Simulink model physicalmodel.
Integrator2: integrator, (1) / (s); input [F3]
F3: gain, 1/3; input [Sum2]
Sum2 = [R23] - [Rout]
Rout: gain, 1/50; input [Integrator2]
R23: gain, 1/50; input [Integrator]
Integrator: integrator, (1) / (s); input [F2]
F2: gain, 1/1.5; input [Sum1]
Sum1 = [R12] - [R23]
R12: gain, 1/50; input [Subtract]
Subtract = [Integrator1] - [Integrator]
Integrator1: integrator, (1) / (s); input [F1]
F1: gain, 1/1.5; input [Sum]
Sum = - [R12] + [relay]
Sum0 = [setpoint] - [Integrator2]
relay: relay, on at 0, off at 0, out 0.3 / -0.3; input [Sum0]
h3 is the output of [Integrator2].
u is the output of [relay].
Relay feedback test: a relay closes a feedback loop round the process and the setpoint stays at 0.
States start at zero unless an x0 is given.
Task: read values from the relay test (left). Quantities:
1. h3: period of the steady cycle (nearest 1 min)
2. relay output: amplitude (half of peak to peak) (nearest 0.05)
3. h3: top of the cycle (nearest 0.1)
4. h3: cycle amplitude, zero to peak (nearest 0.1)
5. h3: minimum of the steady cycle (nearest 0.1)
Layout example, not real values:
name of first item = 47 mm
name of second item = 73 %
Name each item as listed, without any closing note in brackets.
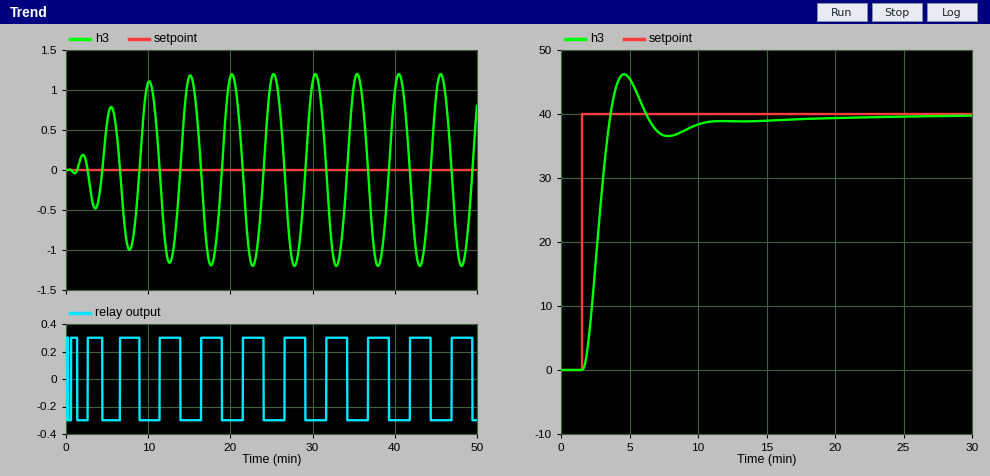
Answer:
h3: period of the steady cycle = 5 min
relay output: amplitude (half of peak to peak) = 0.30
h3: top of the cycle = 1.2
h3: cycle amplitude, zero to peak = 1.2
h3: minimum of the steady cycle = -1.2
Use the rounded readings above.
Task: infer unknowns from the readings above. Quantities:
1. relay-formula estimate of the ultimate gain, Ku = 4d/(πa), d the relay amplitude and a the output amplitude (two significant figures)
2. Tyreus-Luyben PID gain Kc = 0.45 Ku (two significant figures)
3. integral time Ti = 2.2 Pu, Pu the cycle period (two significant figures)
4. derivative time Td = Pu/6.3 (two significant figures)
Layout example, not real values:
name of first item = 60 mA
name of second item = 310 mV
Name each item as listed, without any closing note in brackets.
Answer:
relay-formula estimate of the ultimate gain, Ku = 4d/(πa), d the relay amplitude and a the output amplitude = 0.32
Tyreus-Luyben PID gain Kc = 0.45 Ku = 0.14
integral time Ti = 2.2 Pu, Pu the cycle period = 11 min
derivative time Td = Pu/6.3 = 0.79 min
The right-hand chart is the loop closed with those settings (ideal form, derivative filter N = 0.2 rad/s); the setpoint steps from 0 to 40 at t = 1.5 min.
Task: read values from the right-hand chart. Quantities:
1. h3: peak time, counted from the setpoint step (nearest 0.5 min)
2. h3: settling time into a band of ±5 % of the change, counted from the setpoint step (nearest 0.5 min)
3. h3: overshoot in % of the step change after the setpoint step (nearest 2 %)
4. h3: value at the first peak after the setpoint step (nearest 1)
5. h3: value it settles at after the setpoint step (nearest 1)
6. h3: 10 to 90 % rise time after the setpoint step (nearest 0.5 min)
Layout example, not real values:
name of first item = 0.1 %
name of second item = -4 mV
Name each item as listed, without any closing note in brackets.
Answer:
h3: peak time, counted from the setpoint step = 3.0 min
h3: settling time into a band of ±5 % of the change, counted from the setpoint step = 8.0 min
h3: overshoot in % of the step change after the setpoint step = 16 %
h3: value at the first peak after the setpoint step = 46
h3: value it settles at after the setpoint step = 40
h3: 10 to 90 % rise time after the setpoint step = 1.5 min
